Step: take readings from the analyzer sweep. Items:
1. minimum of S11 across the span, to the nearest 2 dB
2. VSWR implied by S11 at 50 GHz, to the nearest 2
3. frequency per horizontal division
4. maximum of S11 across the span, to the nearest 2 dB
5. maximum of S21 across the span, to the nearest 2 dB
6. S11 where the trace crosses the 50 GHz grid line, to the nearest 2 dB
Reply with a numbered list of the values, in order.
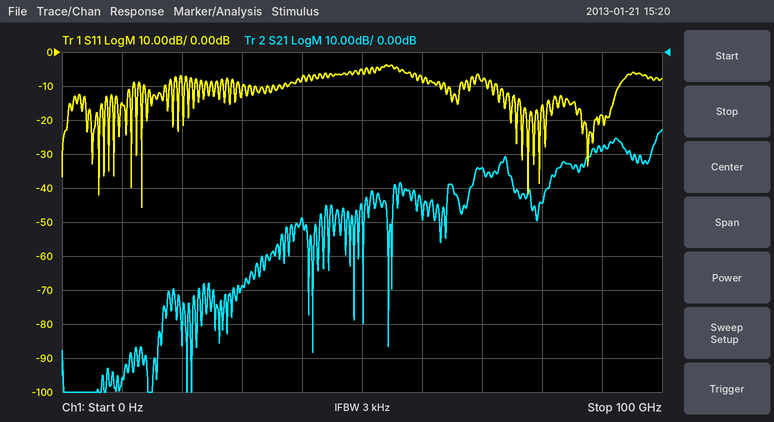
1. -46 dB
2. 4
3. 10 GHz
4. -4 dB
5. -22 dB
6. -6 dB
